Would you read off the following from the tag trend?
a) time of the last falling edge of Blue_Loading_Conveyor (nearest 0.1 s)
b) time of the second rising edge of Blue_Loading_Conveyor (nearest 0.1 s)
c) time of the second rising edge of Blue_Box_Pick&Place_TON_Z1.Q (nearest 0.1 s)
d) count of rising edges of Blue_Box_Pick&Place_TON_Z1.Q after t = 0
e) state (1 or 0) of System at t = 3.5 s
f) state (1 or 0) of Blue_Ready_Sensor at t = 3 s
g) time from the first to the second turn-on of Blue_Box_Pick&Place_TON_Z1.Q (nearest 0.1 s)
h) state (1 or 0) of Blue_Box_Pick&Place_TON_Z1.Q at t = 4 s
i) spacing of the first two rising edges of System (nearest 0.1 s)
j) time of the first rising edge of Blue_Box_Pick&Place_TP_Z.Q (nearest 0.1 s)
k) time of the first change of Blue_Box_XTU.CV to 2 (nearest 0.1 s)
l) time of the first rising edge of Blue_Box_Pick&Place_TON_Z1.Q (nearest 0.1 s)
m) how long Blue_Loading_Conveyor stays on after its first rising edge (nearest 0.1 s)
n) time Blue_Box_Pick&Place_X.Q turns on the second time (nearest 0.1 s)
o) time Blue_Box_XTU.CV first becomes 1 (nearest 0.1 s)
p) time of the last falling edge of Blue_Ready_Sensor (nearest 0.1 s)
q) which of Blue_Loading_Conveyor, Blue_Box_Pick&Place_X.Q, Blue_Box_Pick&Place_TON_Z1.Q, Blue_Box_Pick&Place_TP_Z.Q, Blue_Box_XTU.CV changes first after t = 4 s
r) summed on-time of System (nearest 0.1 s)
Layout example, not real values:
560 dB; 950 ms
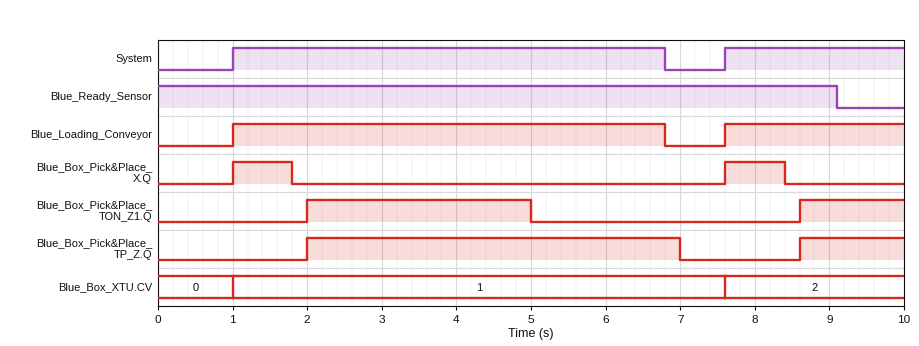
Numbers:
6.8 s; 7.6 s; 8.6 s; 2; 1; 1; 6.6 s; 1; 6.6 s; 2.0 s; 7.6 s; 2.0 s; 5.8 s; 7.6 s; 1.0 s; 9.1 s; Blue_Box_Pick&Place_TON_Z1.Q; 8.2 s
